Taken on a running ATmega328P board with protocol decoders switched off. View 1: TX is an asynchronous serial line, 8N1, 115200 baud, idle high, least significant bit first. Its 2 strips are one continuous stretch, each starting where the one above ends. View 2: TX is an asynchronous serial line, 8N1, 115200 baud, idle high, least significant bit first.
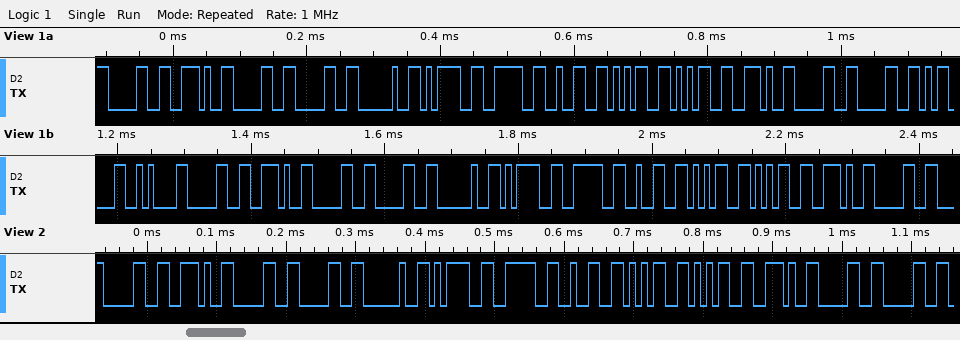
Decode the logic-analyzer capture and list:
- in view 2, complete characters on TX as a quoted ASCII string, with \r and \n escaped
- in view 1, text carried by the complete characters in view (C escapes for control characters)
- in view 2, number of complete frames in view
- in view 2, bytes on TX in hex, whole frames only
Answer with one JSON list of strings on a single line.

["\"0.00 =>255.00\"", "\"0.00 =>255.00\\r\\n0.00 =>255.0\"", "13", "30 2E 30 30 20 3D 3E 32 35 35 2E 30 30"]
